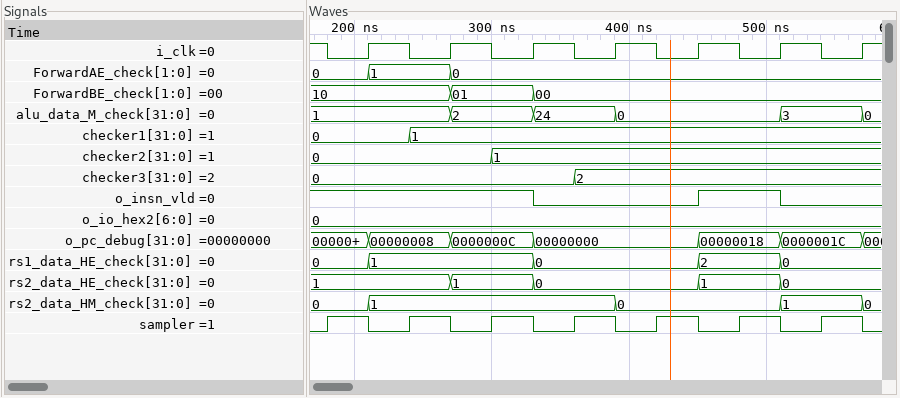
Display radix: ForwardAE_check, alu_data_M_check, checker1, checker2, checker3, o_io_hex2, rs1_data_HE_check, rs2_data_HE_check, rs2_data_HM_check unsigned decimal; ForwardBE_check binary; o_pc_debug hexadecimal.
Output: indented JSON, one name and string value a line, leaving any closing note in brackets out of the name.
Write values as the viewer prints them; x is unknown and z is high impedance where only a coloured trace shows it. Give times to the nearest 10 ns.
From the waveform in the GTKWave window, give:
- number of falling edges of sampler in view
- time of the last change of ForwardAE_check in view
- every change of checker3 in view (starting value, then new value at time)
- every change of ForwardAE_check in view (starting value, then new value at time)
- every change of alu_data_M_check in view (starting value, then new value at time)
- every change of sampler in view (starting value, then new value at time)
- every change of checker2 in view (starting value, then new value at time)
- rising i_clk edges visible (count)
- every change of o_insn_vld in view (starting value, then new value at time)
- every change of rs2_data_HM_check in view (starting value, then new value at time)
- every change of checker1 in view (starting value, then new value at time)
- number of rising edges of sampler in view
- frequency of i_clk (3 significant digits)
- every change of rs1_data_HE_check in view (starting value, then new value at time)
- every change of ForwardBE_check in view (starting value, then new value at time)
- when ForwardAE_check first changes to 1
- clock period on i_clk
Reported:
{
  "number of falling edges of sampler in view": "7",
  "time of the last change of ForwardAE_check in view": "270 ns",
  "every change of checker3 in view": "0, 2 at 360 ns",
  "every change of ForwardAE_check in view": "0, 1 at 210 ns, 0 at 270 ns",
  "every change of alu_data_M_check in view": "1, 2 at 270 ns, 24 at 330 ns, 0 at 390 ns, 3 at 510 ns, 0 at 570 ns",
  "every change of sampler in view": "0, 1 at 180 ns, 0 at 210 ns, 1 at 240 ns, 0 at 270 ns, 1 at 300 ns, 0 at 330 ns, 1 at 360 ns, 0 at 390 ns, 1 at 420 ns, 0 at 450 ns, 1 at 480 ns, 0 at 510 ns, 1 at 540 ns, 0 at 570 ns",
  "every change of checker2 in view": "0, 1 at 300 ns",
  "rising i_clk edges visible": "7",
  "every change of o_insn_vld in view": "1, 0 at 330 ns, 1 at 450 ns, 0 at 510 ns",
  "every change of rs2_data_HM_check in view": "0, 1 at 210 ns, 0 at 390 ns, 1 at 510 ns, 0 at 570 ns",
  "every change of checker1 in view": "0, 1 at 240 ns",
  "number of rising edges of sampler in view": "7",
  "frequency of i_clk": "16.7 MHz",
  "every change of rs1_data_HE_check in view": "0, 1 at 210 ns, 0 at 330 ns, 2 at 450 ns, 0 at 510 ns",
  "every change of ForwardBE_check in view": "10, 01 at 270 ns, 00 at 330 ns",
  "when ForwardAE_check first changes to 1": "210 ns",
  "clock period on i_clk": "60 ns"
}
